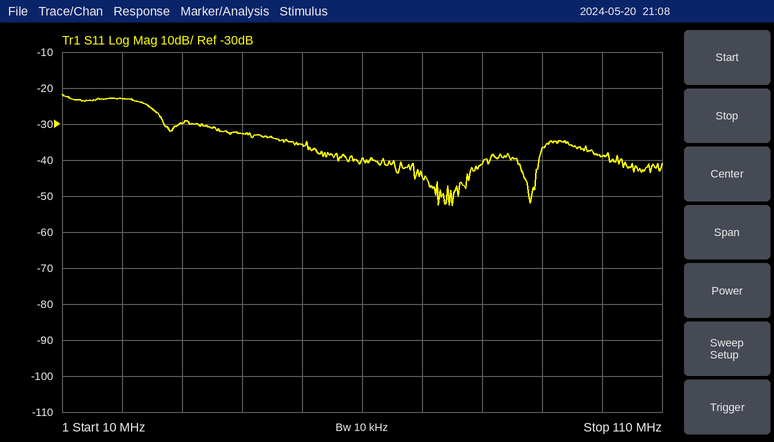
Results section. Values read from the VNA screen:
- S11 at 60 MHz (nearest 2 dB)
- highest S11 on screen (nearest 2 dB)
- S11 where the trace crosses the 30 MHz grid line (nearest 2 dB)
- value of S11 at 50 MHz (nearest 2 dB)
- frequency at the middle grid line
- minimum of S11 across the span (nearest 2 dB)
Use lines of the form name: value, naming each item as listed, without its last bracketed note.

S11 at 60 MHz: -40 dB
highest S11 on screen: -22 dB
S11 where the trace crosses the 30 MHz grid line: -30 dB
value of S11 at 50 MHz: -36 dB
frequency at the middle grid line: 60 MHz
minimum of S11 across the span: -52 dB
